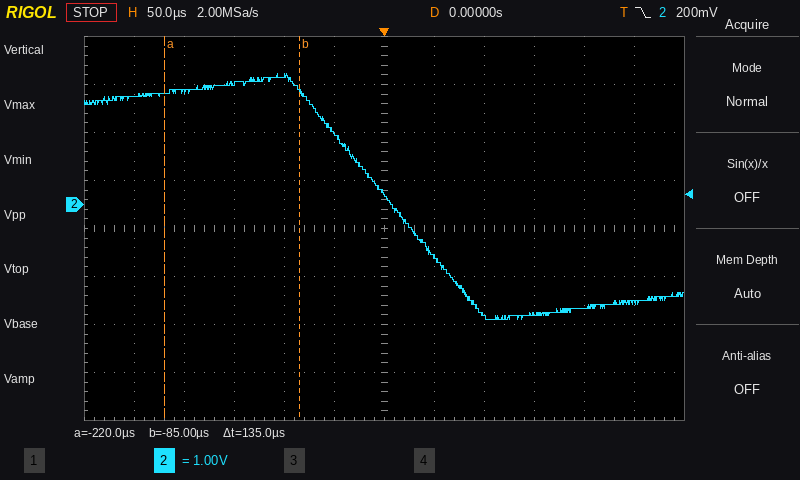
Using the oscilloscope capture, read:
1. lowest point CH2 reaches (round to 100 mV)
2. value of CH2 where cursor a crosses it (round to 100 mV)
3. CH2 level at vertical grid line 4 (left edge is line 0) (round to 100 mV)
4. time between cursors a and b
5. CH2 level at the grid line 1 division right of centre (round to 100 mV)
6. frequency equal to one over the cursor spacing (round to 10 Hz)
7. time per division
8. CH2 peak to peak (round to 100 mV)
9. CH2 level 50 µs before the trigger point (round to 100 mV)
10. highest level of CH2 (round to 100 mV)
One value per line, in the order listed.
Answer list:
-2.4 V
2.3 V
2.7 V
135 µs
-1.1 V
7.41 kHz
50 µs
5.1 V
1.5 V
2.7 V
